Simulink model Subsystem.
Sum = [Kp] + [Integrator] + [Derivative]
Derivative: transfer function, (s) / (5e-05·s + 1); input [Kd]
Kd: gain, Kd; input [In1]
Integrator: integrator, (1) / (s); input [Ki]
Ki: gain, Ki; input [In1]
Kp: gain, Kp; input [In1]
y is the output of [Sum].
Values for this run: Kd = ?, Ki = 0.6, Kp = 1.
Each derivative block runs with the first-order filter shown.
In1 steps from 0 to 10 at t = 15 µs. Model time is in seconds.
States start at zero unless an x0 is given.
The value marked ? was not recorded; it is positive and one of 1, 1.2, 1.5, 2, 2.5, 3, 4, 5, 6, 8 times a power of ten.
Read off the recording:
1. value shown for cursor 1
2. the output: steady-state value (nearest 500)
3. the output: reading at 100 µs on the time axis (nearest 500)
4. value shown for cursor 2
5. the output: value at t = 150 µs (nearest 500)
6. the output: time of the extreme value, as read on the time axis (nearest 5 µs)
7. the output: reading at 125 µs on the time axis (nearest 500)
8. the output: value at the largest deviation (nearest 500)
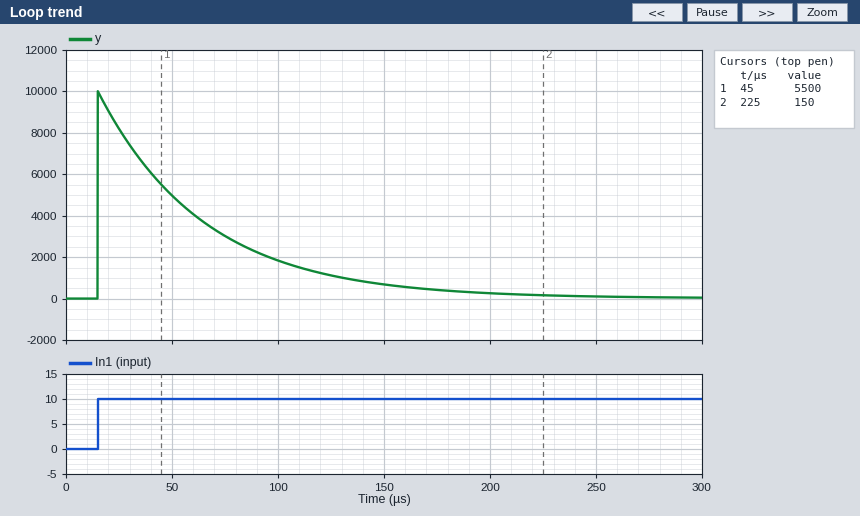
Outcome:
5500
0
2000
150
500
15 µs
1000
10000
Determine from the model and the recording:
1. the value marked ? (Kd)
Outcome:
0.05
